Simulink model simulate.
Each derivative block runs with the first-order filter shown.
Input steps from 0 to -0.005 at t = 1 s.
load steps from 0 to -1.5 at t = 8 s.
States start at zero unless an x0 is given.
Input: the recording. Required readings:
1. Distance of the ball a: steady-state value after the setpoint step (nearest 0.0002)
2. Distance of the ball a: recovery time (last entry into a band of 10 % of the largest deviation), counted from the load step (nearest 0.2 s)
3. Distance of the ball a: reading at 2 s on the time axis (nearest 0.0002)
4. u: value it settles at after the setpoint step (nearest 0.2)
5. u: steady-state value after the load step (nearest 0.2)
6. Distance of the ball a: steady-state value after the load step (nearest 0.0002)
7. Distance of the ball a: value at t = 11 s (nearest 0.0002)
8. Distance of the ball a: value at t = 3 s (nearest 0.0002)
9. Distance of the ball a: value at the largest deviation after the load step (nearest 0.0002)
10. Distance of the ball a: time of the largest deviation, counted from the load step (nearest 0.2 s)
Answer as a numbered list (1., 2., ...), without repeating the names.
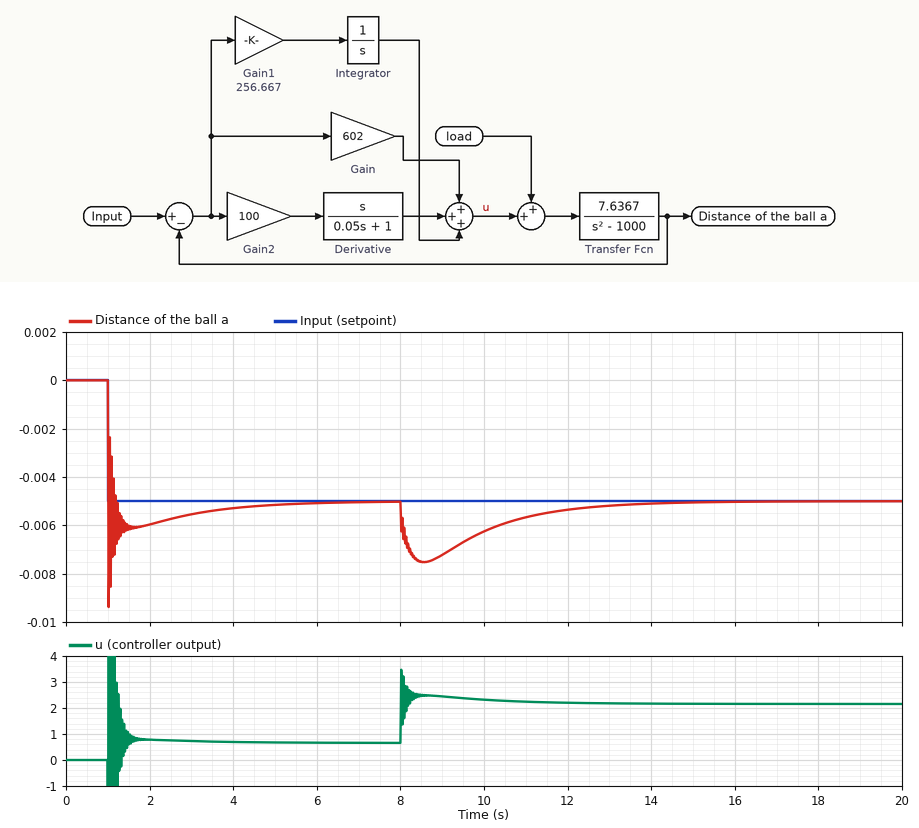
1. -0.0050
2. 4.6 s
3. -0.0060
4. 0.6
5. 2.2
6. -0.0050
7. -0.0056
8. -0.0056
9. -0.0076
10. 0.6 s
